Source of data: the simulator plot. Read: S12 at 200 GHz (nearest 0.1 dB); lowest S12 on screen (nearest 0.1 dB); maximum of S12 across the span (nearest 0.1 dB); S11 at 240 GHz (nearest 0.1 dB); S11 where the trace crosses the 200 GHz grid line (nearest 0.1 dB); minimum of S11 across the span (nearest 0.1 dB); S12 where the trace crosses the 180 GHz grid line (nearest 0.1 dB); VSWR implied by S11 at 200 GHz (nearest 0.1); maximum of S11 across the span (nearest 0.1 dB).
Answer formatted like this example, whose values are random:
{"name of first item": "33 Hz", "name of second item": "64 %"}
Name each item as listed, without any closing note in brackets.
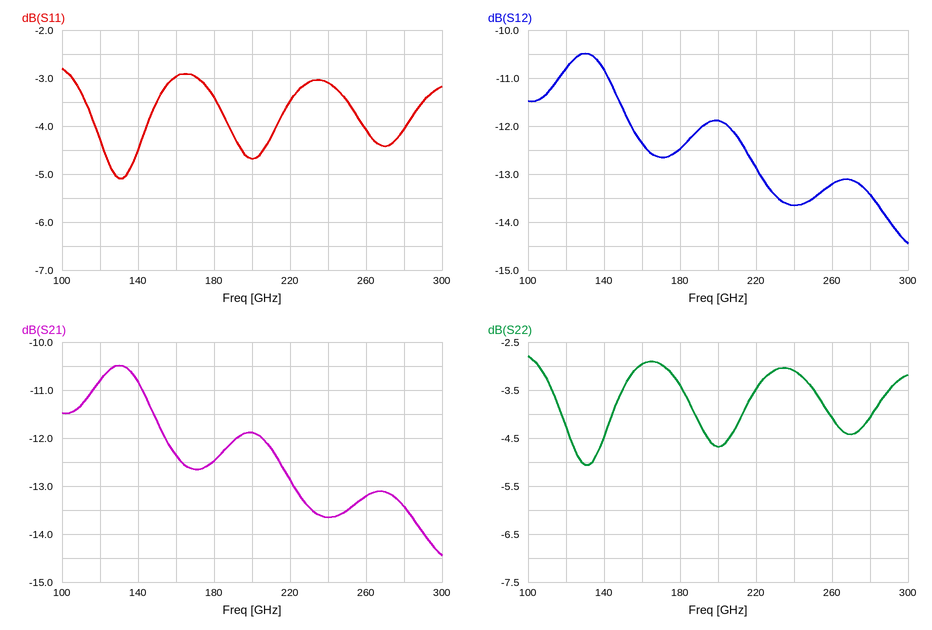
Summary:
{"S12 at 200 GHz": "-11.9 dB", "lowest S12 on screen": "-14.4 dB", "maximum of S12 across the span": "-10.5 dB", "S11 at 240 GHz": "-3.1 dB", "S11 where the trace crosses the 200 GHz grid line": "-4.7 dB", "minimum of S11 across the span": "-5.1 dB", "S12 where the trace crosses the 180 GHz grid line": "-12.5 dB", "VSWR implied by S11 at 200 GHz": "3.8", "maximum of S11 across the span": "-2.8 dB"}
